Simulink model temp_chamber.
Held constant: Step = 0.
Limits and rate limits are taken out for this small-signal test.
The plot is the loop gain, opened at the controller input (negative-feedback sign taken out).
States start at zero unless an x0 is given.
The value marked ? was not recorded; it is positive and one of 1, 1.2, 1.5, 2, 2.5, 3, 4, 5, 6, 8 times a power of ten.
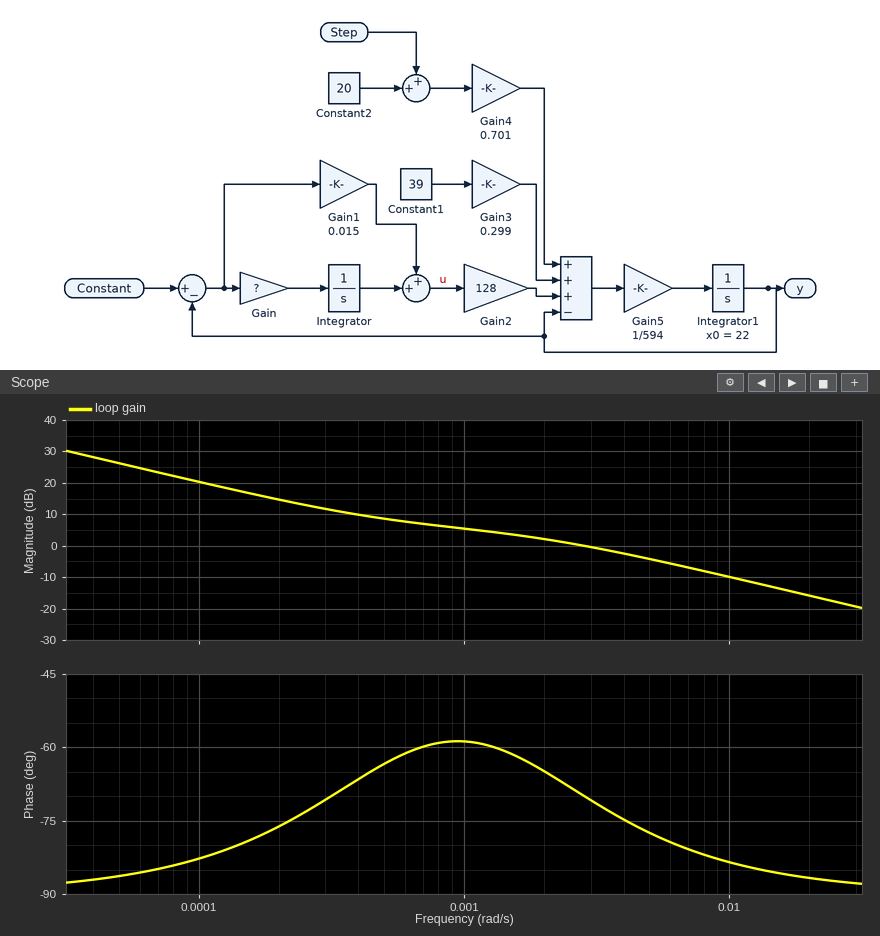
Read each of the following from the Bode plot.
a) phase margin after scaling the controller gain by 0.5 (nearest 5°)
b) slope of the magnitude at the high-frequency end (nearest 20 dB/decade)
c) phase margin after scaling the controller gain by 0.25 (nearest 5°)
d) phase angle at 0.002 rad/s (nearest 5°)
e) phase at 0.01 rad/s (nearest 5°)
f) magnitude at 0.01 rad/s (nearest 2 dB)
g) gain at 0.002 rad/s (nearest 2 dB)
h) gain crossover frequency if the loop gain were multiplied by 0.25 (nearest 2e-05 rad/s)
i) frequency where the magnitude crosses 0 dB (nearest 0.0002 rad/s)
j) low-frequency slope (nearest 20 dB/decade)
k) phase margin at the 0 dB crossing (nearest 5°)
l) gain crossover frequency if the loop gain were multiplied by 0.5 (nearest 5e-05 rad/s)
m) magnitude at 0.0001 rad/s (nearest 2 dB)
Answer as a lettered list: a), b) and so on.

a) 120°
b) -20 dB/decade
c) 110°
d) -65°
e) -85°
f) -10 dB
g) 2 dB
h) 0.00028 rad/s
i) 0.0028 rad/s
j) -20 dB/decade
k) 110°
l) 0.00085 rad/s
m) 20 dB
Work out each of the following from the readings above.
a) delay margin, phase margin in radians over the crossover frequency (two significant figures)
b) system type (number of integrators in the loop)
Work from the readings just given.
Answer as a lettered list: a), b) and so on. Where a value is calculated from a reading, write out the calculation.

a) 110 × π / 180 / 0.0028 = 690 s
b) 1
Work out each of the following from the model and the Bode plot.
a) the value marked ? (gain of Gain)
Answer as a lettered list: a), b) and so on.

a) 8e-06
